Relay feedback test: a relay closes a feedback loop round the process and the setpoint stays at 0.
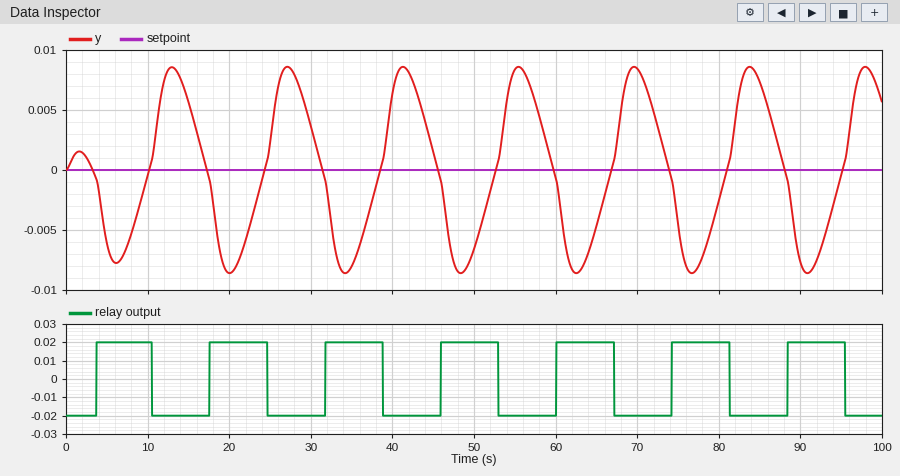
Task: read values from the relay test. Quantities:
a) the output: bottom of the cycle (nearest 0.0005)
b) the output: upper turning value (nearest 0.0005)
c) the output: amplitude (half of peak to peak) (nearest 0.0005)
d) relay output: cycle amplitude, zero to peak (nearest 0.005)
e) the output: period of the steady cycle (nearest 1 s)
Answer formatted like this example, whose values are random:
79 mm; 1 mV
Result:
-0.0085; 0.0085; 0.0085; 0.020; 14 s
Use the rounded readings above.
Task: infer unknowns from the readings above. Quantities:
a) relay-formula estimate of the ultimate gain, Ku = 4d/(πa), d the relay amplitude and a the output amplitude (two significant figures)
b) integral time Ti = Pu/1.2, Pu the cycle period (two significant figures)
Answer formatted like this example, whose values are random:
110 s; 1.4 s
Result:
3.0; 12 s
